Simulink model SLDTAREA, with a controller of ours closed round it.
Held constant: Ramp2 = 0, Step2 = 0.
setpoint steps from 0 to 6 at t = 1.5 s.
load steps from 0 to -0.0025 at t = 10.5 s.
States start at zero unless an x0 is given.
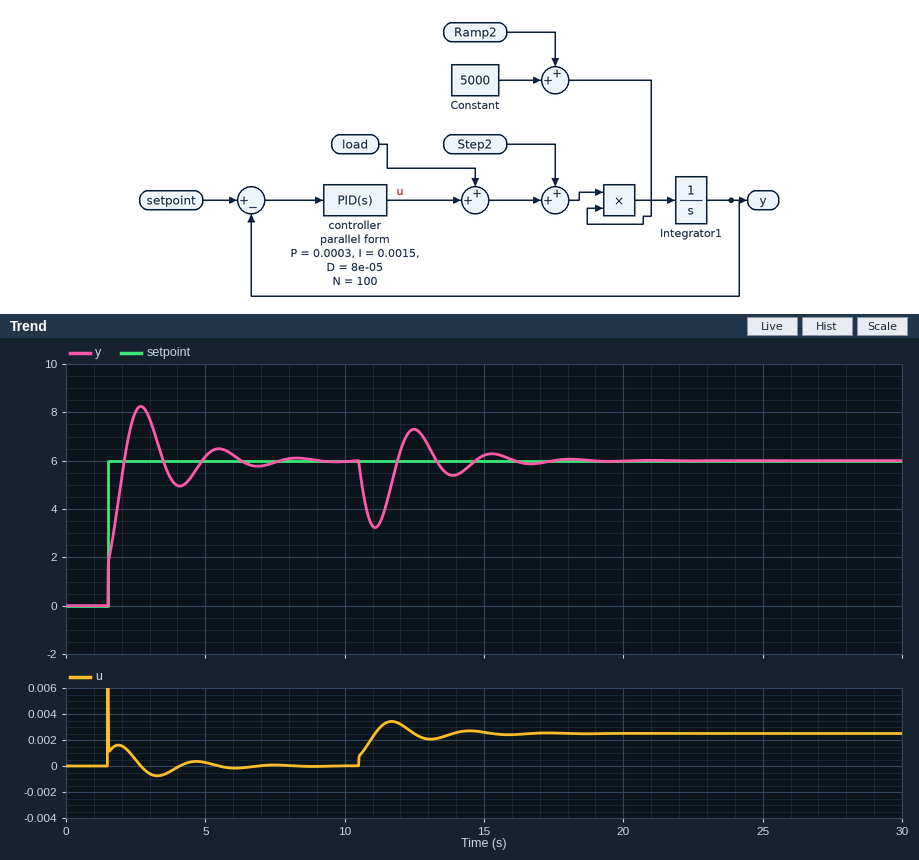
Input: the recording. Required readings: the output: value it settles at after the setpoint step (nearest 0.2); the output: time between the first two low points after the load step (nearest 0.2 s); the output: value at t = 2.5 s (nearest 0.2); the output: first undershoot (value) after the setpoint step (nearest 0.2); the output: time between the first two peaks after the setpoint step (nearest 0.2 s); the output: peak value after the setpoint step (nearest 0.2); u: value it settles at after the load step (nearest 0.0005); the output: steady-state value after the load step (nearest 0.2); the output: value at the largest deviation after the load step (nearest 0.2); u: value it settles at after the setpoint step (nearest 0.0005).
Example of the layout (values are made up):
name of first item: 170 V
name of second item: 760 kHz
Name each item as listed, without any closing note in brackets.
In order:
the output: value it settles at after the setpoint step: 6.0
the output: time between the first two low points after the load step: 2.8 s
the output: value at t = 2.5 s: 8.0
the output: first undershoot (value) after the setpoint step: 5.0
the output: time between the first two peaks after the setpoint step: 2.8 s
the output: peak value after the setpoint step: 8.2
u: value it settles at after the load step: 0.0025
the output: steady-state value after the load step: 6.0
the output: value at the largest deviation after the load step: 3.2
u: value it settles at after the setpoint step: 0.0000
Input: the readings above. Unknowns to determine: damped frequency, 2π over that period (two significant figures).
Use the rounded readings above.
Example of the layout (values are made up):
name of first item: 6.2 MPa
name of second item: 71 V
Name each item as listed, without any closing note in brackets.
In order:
damped frequency, 2π over that period: 2.2 rad/s
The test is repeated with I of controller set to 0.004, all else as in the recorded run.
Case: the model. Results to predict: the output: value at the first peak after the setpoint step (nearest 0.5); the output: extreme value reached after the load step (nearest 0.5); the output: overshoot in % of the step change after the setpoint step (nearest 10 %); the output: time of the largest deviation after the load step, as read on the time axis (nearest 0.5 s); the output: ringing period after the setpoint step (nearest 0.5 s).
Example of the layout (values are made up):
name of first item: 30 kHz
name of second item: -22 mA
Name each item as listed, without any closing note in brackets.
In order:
the output: value at the first peak after the setpoint step: 9.0
the output: extreme value reached after the load step: 4.0
the output: overshoot in % of the step change after the setpoint step: 50 %
the output: time of the largest deviation after the load step, as read on the time axis: 11.0 s
the output: ringing period after the setpoint step: 1.5 s
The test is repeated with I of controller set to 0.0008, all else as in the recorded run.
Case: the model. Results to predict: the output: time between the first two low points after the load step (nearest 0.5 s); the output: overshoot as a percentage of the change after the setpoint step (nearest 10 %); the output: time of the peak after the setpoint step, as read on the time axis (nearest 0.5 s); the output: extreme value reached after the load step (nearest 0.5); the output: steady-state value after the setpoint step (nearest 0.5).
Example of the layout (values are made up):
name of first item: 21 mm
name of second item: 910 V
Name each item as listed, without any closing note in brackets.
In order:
the output: time between the first two low points after the load step: 4.0 s
the output: overshoot as a percentage of the change after the setpoint step: 30 %
the output: time of the peak after the setpoint step, as read on the time axis: 3.0 s
the output: extreme value reached after the load step: 2.5
the output: steady-state value after the setpoint step: 6.0
